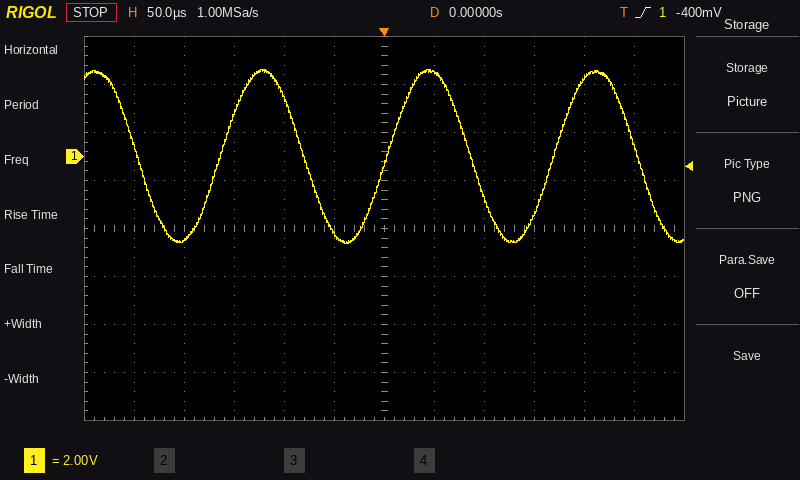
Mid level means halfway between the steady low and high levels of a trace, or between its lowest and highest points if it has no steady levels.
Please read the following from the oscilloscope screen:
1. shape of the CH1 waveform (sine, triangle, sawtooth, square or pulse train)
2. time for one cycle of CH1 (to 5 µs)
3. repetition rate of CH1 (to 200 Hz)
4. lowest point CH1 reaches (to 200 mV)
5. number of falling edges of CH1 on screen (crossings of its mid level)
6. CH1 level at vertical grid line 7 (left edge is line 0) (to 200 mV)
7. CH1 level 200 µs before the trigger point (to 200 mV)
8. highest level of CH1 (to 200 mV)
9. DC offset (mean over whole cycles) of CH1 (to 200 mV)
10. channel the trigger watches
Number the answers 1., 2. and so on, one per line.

1. sine
2. 165 µs
3. 6.0 kHz
4. -3.6 V
5. 4
6. 3.4 V
7. -3.4 V
8. 3.6 V
9. 0.0 V
10. CH1
